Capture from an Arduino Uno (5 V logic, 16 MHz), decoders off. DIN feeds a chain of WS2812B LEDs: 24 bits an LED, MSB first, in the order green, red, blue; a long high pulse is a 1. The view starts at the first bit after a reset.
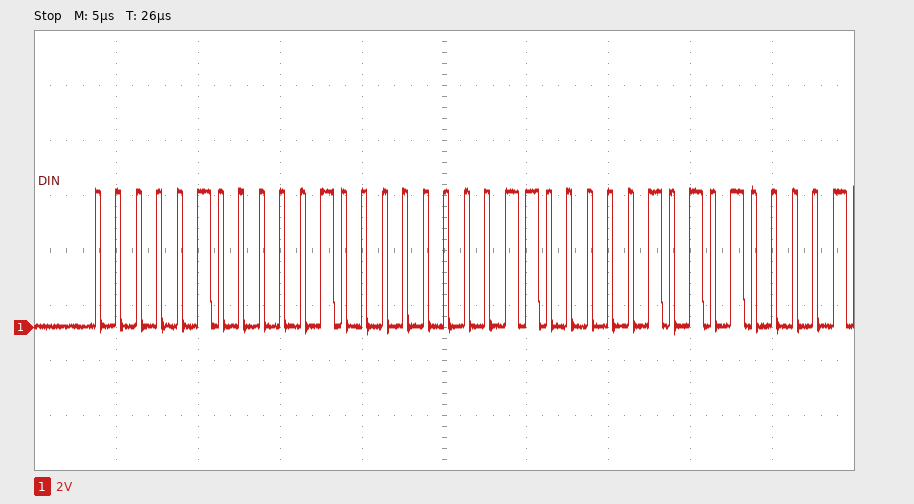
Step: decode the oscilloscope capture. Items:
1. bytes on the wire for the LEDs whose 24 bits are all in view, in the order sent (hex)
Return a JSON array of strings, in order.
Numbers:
["04 10 0C"]
